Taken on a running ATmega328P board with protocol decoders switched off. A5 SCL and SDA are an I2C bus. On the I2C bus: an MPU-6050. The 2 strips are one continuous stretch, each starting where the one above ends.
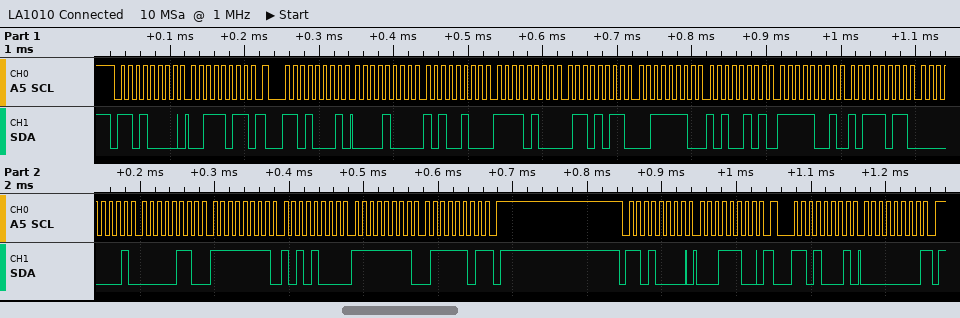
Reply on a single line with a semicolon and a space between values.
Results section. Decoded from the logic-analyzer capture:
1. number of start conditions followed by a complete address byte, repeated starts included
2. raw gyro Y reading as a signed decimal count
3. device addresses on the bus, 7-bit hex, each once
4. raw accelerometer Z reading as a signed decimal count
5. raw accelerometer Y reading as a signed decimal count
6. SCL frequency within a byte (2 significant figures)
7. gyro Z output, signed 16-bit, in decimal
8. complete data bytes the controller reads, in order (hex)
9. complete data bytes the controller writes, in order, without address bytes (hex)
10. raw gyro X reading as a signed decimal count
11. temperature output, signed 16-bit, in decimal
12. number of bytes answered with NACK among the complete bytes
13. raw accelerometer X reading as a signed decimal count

4; -88; 0x68; 16037; -2965; 100 kHz; -131; 08 A4 F4 6B 3E A5 F9 BB 01 06 FF A8 FF 7D 00; 3B 1C; 262; -1605; 2; 2212
